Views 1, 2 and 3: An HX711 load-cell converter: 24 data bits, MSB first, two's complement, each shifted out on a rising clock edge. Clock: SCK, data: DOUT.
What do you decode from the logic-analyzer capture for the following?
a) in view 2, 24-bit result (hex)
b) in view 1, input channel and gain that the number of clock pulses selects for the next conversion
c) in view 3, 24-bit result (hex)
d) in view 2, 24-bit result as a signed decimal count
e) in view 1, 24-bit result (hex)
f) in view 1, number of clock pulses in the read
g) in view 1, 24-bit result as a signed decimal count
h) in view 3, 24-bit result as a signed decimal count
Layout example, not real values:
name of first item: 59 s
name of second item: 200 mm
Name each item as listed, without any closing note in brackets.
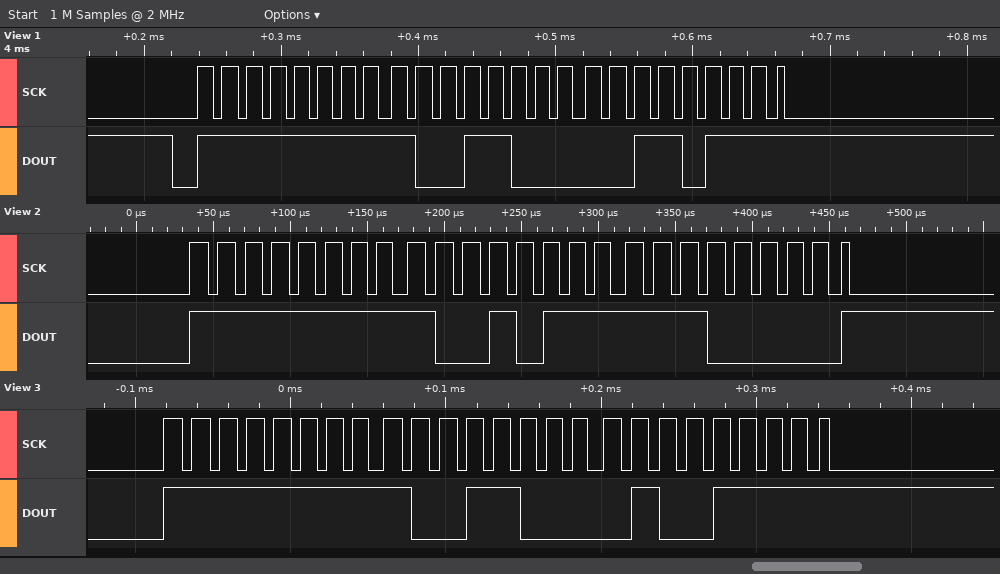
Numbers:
in view 2, 24-bit result: 0xFF97E0
in view 1, input channel and gain that the number of clock pulses selects for the next conversion: channel A, gain 128
in view 3, 24-bit result: 0xFF984F
in view 2, 24-bit result as a signed decimal count: -26656
in view 1, 24-bit result: 0xFF9837
in view 1, number of clock pulses in the read: 25
in view 1, 24-bit result as a signed decimal count: -26569
in view 3, 24-bit result as a signed decimal count: -26545
